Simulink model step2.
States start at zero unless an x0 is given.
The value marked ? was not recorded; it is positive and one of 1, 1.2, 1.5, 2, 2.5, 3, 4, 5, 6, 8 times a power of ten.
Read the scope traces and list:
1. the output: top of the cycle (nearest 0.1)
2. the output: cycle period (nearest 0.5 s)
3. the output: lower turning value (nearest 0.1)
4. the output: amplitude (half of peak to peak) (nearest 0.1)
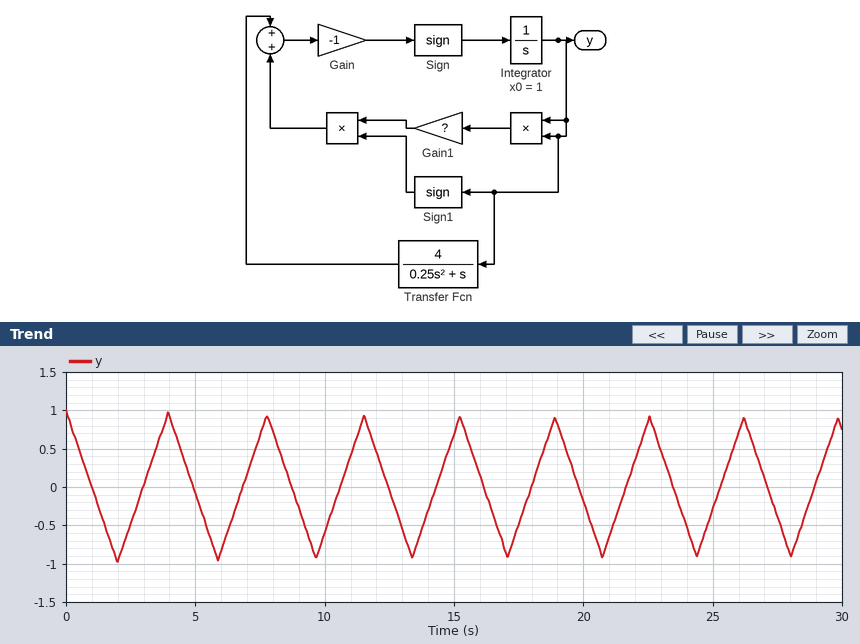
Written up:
0.9
3.5 s
-0.9
0.9
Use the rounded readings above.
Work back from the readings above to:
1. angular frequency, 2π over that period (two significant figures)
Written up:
1.8 rad/s
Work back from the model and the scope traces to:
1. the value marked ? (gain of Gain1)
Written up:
0.8
